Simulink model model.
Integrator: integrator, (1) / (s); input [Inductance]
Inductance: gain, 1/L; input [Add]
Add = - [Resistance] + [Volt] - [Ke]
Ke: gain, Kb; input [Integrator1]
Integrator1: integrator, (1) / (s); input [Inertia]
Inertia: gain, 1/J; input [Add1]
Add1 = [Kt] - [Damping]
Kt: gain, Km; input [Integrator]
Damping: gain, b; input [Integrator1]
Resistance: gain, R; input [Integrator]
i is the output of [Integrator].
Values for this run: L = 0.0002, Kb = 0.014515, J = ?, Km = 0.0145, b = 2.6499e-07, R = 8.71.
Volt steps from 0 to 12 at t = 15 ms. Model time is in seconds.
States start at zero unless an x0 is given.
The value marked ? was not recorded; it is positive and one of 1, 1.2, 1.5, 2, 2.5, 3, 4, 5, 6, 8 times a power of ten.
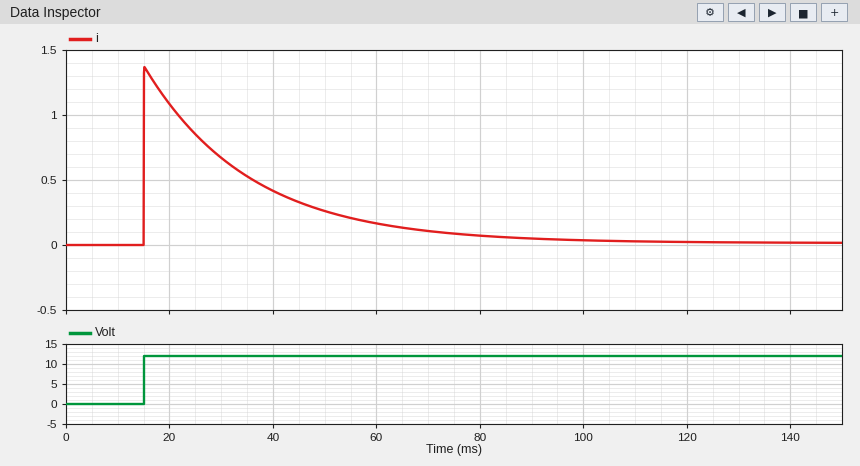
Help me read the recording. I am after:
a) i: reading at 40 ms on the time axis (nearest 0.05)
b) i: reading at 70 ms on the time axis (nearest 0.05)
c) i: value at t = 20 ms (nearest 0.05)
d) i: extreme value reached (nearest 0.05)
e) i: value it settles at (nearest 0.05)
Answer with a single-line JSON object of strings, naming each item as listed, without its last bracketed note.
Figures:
{"i: reading at 40 ms on the time axis": "0.40", "i: reading at 70 ms on the time axis": "0.10", "i: value at t = 20 ms": "1.10", "i: extreme value reached": "1.35", "i: value it settles at": "0.00"}
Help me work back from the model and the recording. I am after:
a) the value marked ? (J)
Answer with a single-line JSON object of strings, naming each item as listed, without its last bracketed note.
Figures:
{"the value marked ?": "5e-07"}
